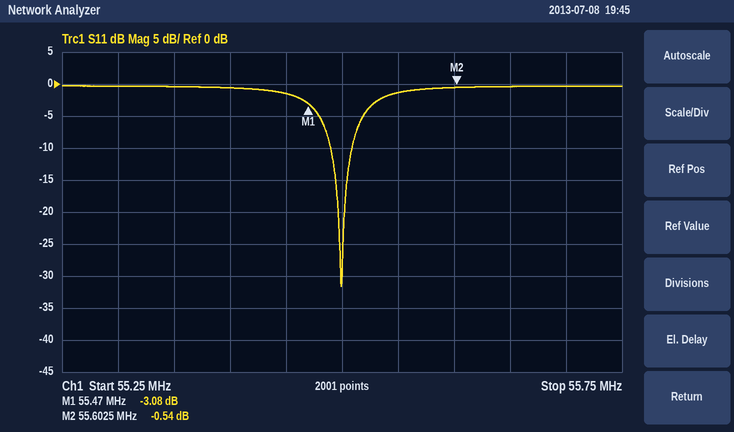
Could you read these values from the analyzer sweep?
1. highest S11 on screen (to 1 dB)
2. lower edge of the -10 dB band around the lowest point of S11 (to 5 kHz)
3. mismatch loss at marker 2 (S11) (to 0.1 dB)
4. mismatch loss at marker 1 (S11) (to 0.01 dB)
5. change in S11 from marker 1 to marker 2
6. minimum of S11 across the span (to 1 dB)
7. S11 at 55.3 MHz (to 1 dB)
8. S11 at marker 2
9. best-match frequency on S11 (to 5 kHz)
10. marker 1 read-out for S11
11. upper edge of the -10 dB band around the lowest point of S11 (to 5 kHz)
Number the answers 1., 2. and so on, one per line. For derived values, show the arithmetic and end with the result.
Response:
1. 0 dB
2. 55.490 MHz
3. −10 log10(1 − 10^(-0.54/10)) ≈ 9.3 dB
4. −10 log10(1 − 10^(-3.08/10)) ≈ 2.94 dB
5. -0.54 − (-3.08) = 2.54 dB
6. -32 dB
7. 0 dB
8. -0.54 dB
9. 55.500 MHz
10. -3.08 dB
11. 55.510 MHz
